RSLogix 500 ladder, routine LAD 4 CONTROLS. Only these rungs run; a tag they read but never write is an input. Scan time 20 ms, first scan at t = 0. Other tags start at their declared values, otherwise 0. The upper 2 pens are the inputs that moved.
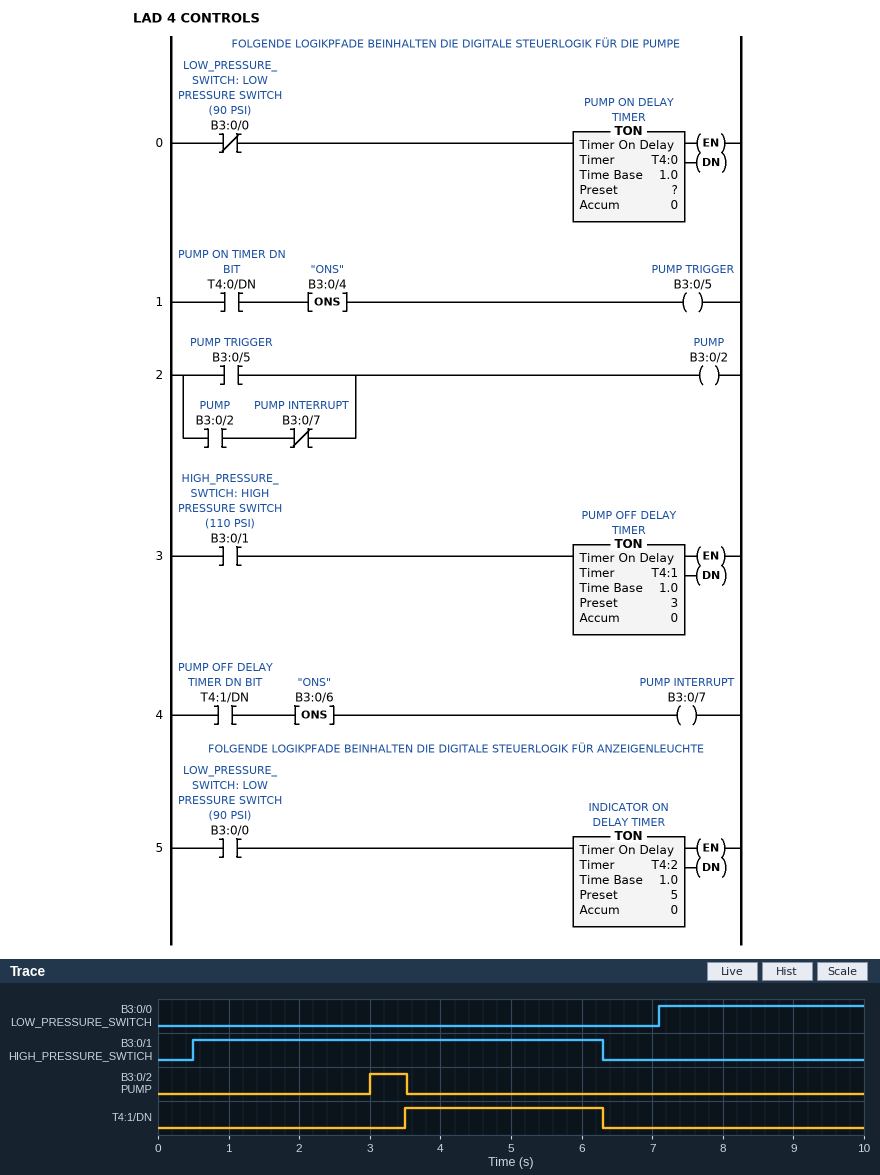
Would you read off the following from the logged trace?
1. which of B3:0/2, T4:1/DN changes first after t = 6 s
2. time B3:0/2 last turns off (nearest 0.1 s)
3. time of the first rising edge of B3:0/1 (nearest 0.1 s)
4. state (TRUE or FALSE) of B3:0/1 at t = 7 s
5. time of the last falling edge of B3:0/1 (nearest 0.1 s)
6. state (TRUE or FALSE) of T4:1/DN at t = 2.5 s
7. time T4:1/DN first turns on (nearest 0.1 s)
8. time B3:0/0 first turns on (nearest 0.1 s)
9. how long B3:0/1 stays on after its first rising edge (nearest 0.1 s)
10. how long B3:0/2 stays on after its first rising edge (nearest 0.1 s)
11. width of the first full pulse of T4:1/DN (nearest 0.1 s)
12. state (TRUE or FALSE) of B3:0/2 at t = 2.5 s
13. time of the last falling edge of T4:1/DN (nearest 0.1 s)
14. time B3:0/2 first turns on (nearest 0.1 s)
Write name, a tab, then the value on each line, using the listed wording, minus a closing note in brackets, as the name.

which of B3:0/2, T4:1/DN changes first after t = 6 s	T4:1/DN
time B3:0/2 last turns off	3.5 s
time of the first rising edge of B3:0/1	0.5 s
state (TRUE or FALSE) of B3:0/1 at t = 7 s	FALSE
time of the last falling edge of B3:0/1	6.3 s
state (TRUE or FALSE) of T4:1/DN at t = 2.5 s	FALSE
time T4:1/DN first turns on	3.5 s
time B3:0/0 first turns on	7.1 s
how long B3:0/1 stays on after its first rising edge	5.8 s
how long B3:0/2 stays on after its first rising edge	0.5 s
width of the first full pulse of T4:1/DN	2.8 s
state (TRUE or FALSE) of B3:0/2 at t = 2.5 s	FALSE
time of the last falling edge of T4:1/DN	6.3 s
time B3:0/2 first turns on	3.0 s
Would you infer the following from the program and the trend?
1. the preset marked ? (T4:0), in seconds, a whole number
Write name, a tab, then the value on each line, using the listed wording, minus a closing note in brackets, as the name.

the preset marked ? (T4:0), in seconds, a whole number	3 s
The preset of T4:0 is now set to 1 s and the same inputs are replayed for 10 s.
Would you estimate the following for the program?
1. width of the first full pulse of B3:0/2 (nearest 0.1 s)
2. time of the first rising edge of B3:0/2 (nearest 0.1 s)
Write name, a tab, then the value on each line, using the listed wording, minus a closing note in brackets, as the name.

width of the first full pulse of B3:0/2	2.5 s
time of the first rising edge of B3:0/2	1.0 s
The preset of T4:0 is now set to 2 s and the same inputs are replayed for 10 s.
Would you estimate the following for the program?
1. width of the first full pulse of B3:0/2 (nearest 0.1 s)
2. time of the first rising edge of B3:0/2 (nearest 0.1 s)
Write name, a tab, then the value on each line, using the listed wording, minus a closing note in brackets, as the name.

width of the first full pulse of B3:0/2	1.5 s
time of the first rising edge of B3:0/2	2.0 s
